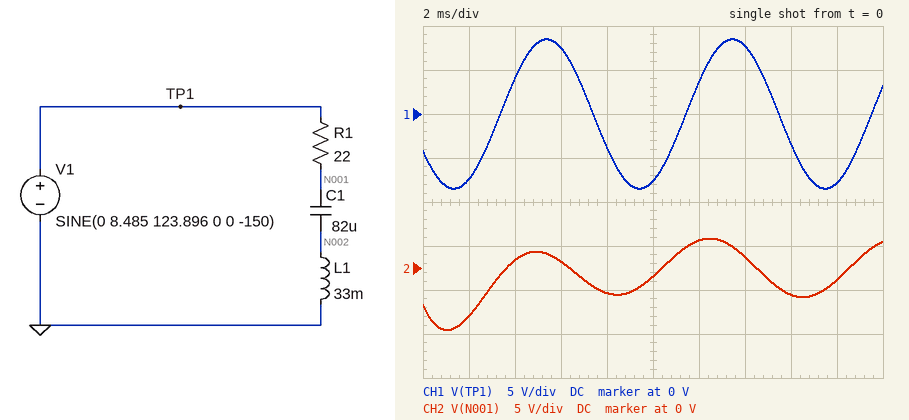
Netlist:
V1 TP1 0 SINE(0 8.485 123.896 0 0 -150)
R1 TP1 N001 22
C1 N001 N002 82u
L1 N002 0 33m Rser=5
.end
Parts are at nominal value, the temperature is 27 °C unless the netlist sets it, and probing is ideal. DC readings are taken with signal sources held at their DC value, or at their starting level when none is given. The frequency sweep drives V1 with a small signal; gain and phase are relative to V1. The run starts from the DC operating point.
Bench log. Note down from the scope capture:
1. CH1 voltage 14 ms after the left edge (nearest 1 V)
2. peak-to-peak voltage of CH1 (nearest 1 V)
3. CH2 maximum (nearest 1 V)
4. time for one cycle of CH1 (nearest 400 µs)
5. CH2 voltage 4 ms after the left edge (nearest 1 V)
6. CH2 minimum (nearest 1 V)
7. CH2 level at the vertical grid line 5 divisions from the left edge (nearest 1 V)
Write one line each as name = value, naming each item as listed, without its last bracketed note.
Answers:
CH1 voltage 14 ms after the left edge = 8 V
peak-to-peak voltage of CH1 = 17 V
CH2 maximum = 3 V
time for one cycle of CH1 = 8.0 ms
CH2 voltage 4 ms after the left edge = 1 V
CH2 minimum = -7 V
CH2 level at the vertical grid line 5 divisions from the left edge = -1 V
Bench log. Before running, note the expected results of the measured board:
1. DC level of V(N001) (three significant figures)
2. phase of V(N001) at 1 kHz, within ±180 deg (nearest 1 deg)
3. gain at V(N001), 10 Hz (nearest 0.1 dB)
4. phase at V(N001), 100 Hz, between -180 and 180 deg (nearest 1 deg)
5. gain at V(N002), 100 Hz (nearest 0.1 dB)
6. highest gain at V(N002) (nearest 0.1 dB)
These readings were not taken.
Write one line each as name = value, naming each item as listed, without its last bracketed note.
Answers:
DC level of V(N001) = -4.24 V
phase of V(N001) at 1 kHz, within ±180 deg = 6 deg
gain at V(N001), 10 Hz = -0.1 dB
phase at V(N001), 100 Hz, between -180 and 180 deg = 12 deg
gain at V(N002), 100 Hz = -2.1 dB
highest gain at V(N002) = 0.1 dB
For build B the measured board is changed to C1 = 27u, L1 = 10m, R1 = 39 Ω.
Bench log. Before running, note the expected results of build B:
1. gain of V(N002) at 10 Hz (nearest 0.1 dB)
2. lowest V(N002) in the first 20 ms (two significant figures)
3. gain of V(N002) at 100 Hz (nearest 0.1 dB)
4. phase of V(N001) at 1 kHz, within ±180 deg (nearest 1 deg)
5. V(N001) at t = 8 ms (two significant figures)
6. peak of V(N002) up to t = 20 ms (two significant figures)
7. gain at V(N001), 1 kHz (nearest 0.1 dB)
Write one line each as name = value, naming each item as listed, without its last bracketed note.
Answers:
gain of V(N002) at 10 Hz = -41.4 dB
lowest V(N002) in the first 20 ms = -1.3 V
gain of V(N002) at 100 Hz = -18.6 dB
phase of V(N001) at 1 kHz, within ±180 deg = 33 deg
V(N001) at t = 8 ms = 1.4 V
peak of V(N002) up to t = 20 ms = 1.3 V
gain at V(N001), 1 kHz = -2.0 dB
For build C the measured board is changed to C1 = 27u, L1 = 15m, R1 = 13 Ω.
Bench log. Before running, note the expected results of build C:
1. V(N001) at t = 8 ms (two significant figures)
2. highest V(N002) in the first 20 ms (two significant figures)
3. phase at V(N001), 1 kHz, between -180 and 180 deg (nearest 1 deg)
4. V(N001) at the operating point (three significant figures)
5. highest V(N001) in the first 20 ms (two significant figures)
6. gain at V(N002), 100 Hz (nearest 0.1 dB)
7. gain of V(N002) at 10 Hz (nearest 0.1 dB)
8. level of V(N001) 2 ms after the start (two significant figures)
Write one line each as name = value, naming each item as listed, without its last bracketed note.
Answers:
V(N001) at t = 8 ms = -1.1 V
highest V(N002) in the first 20 ms = 3.2 V
phase at V(N001), 1 kHz, between -180 and 180 deg = 8 deg
V(N001) at the operating point = -4.24 V
highest V(N001) in the first 20 ms = 7.7 V
gain at V(N002), 100 Hz = -13.9 dB
gain of V(N002) at 10 Hz = -41.3 dB
level of V(N001) 2 ms after the start = -6.8 V
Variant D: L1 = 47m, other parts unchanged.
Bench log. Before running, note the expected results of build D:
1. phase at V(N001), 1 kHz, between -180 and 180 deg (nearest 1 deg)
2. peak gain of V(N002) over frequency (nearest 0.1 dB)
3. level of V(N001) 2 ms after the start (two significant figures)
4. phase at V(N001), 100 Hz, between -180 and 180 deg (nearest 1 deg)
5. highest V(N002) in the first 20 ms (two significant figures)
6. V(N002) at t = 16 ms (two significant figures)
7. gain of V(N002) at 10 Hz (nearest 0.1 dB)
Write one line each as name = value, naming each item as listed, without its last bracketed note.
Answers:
phase at V(N001), 1 kHz, between -180 and 180 deg = 4 deg
peak gain of V(N002) over frequency = 0.7 dB
level of V(N001) 2 ms after the start = -5.7 V
phase at V(N001), 100 Hz, between -180 and 180 deg = 43 deg
highest V(N002) in the first 20 ms = 9.4 V
V(N002) at t = 16 ms = -8.4 V
gain of V(N002) at 10 Hz = -30.4 dB
